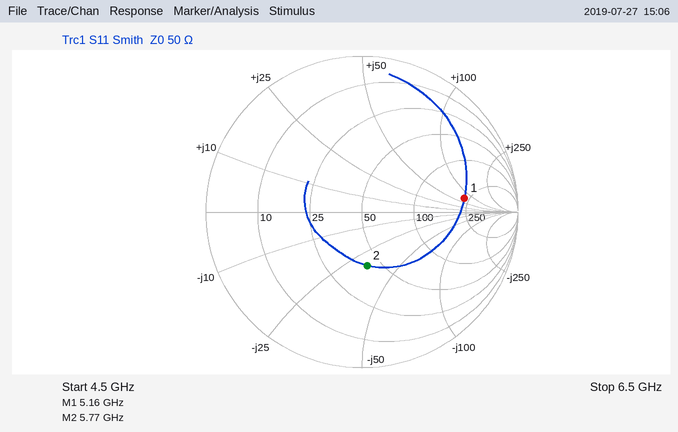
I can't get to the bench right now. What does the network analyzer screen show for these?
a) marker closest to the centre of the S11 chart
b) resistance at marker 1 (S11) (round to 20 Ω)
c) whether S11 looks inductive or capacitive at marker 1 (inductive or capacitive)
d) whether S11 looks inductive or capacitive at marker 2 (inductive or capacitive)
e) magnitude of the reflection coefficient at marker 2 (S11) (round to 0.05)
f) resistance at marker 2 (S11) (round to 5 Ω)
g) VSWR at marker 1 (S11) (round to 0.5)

marker 2
220 Ω
inductive
capacitive
0.35
40 Ω
5.0
